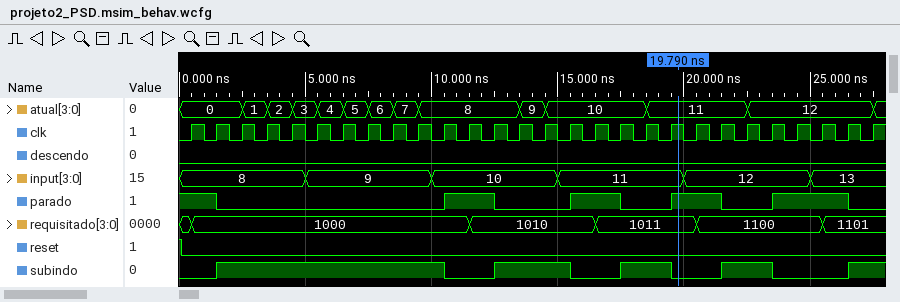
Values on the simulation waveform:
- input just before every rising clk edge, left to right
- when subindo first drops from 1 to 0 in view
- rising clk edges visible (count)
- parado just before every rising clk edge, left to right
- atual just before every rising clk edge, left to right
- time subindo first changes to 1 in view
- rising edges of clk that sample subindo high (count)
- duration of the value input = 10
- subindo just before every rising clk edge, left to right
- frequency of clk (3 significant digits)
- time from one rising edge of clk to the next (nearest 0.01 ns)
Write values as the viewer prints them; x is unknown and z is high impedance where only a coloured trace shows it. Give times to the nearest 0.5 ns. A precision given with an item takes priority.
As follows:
8, 8, 8, 8, 8, 9, 9, 9, 9, 9, 10, 10, 10, 10, 10, 11, 11, 11, 11, 11, 12, 12, 12, 12, 12, 13, 13, 13
10.5 ns
28
1 1 0 0 0 0 0 0 0 0 0 1 1 0 0 0 1 1 0 0 1 1 0 0 1 1 1 0
0, 0, 0, 1, 2, 3, 4, 5, 6, 7, 8, 8, 8, 8, 9, 10, 10, 10, 10, 11, 11, 11, 11, 12, 12, 12, 12, 12
1.5 ns
17
5 ns
0 0 1 1 1 1 1 1 1 1 1 0 0 1 1 1 0 0 1 1 0 0 1 1 0 0 0 1
1.00 GHz
1 ns
